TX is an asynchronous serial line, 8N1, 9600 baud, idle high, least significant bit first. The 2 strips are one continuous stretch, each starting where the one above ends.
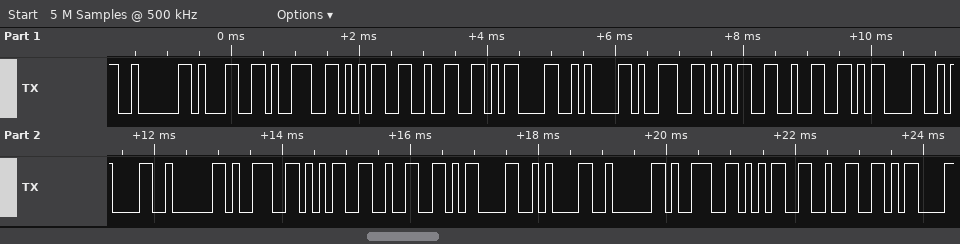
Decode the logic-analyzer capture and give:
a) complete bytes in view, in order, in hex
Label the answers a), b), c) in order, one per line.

a) 02 31 39 35 32 0D 0A 39 35 32 0D 0A 02 39 35 32 0D 0A 02 39 35 32 0D
